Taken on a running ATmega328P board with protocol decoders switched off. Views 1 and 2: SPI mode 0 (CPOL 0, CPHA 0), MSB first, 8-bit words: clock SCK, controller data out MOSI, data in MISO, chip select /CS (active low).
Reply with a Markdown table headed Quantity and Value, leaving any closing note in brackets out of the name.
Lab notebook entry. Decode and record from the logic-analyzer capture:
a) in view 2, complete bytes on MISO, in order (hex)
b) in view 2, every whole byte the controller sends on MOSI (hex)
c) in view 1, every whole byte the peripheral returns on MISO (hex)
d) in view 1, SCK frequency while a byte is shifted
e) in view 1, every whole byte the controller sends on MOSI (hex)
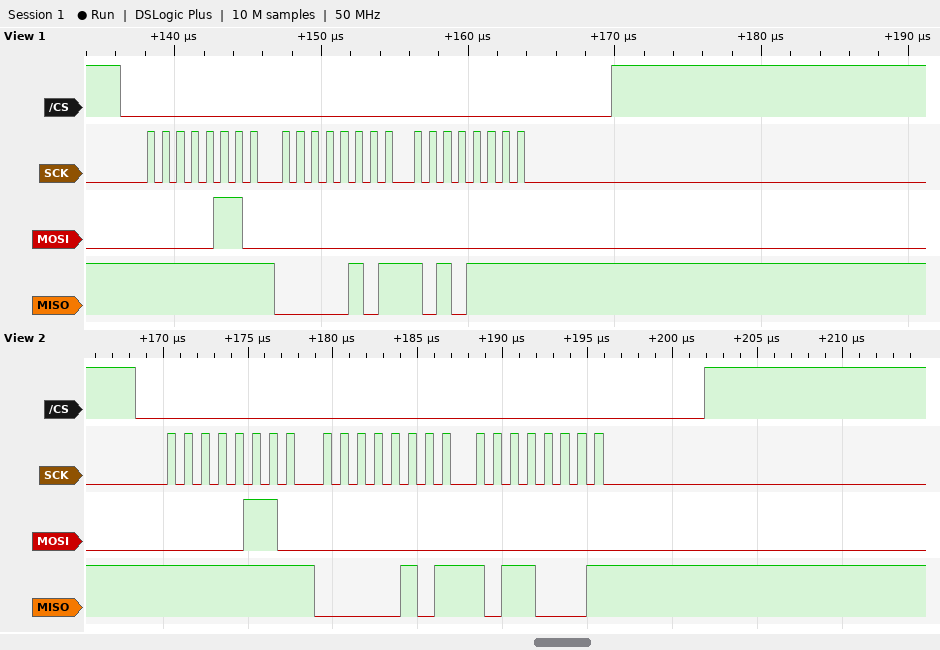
| Quantity | Value |
|---|---|
| in view 2, complete bytes on MISO, in order | FF 05 B1 |
| in view 2, every whole byte the controller sends on MOSI | 06 00 00 |
| in view 1, every whole byte the peripheral returns on MISO | FF 05 AF |
| in view 1, SCK frequency while a byte is shifted | 1 MHz |
| in view 1, every whole byte the controller sends on MOSI | 06 00 00 |
